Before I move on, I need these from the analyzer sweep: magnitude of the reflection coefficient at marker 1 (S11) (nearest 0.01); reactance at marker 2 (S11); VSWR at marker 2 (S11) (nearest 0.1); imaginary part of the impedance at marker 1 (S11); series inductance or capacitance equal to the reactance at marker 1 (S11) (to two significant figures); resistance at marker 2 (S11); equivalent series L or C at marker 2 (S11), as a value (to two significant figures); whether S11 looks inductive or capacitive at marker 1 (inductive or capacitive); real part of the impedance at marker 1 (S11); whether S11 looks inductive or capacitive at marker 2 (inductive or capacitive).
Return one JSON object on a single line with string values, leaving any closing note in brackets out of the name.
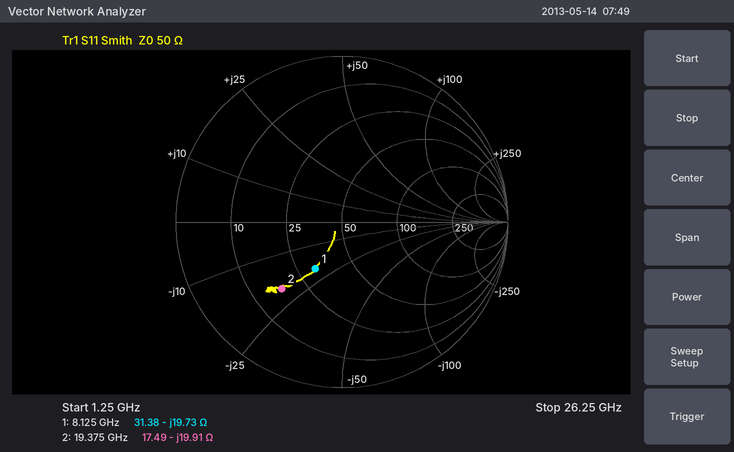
{"magnitude of the reflection coefficient at marker 1 (S11)": "0.32", "reactance at marker 2": "-19.91 Ω", "VSWR at marker 2 (S11)": "3.4", "imaginary part of the impedance at marker 1": "-19.73 Ω", "series inductance or capacitance equal to the reactance at marker 1 (S11)": "990 fF", "resistance at marker 2": "17.49 Ω", "equivalent series L or C at marker 2 (S11), as a value": "410 fF", "whether S11 looks inductive or capacitive at marker 1": "capacitive", "real part of the impedance at marker 1": "31.38 Ω", "whether S11 looks inductive or capacitive at marker 2": "capacitive"}
